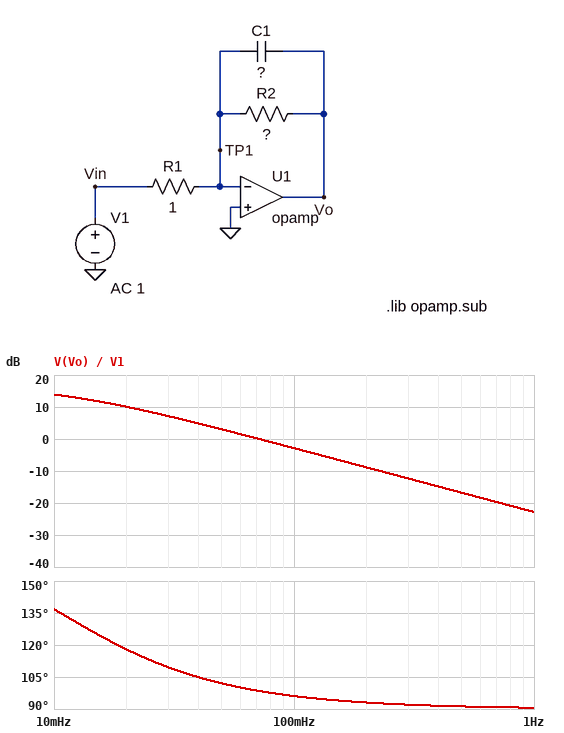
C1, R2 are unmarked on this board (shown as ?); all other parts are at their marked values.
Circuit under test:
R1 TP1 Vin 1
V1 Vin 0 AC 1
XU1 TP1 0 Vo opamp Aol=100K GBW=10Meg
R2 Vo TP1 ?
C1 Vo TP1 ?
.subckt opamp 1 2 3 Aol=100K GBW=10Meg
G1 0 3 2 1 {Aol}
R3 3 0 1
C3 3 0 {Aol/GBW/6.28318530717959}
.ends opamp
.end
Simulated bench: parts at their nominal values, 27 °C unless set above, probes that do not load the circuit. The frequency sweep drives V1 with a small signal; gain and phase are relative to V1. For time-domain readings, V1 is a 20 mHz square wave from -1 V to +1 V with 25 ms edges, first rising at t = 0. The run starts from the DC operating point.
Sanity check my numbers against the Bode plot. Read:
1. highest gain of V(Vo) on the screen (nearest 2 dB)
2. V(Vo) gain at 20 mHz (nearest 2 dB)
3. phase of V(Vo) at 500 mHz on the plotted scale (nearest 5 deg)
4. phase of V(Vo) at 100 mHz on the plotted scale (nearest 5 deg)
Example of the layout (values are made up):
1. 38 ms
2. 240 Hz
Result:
1. 14 dB
2. 10 dB
3. 90 deg
4. 95 deg
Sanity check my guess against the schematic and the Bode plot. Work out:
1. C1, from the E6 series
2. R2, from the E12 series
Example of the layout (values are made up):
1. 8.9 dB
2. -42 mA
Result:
1. 2.2 F
2. 6.8 Ω
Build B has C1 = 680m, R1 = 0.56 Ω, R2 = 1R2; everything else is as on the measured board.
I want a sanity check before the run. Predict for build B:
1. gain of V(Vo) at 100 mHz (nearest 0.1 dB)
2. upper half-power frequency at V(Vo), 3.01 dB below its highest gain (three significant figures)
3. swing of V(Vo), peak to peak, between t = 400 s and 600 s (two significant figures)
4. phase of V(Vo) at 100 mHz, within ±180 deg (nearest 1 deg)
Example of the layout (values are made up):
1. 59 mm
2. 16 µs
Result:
1. 5.6 dB
2. 195 mHz
3. 4.3 V
4. 153 deg
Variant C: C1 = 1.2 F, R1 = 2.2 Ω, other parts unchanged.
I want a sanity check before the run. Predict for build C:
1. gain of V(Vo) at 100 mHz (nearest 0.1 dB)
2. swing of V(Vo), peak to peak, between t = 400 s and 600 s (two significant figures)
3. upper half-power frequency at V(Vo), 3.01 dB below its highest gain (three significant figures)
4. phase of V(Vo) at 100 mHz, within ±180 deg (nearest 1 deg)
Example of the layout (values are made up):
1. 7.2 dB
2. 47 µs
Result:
1. -4.6 dB
2. 5.6 V
3. 19.5 mHz
4. 101 deg
